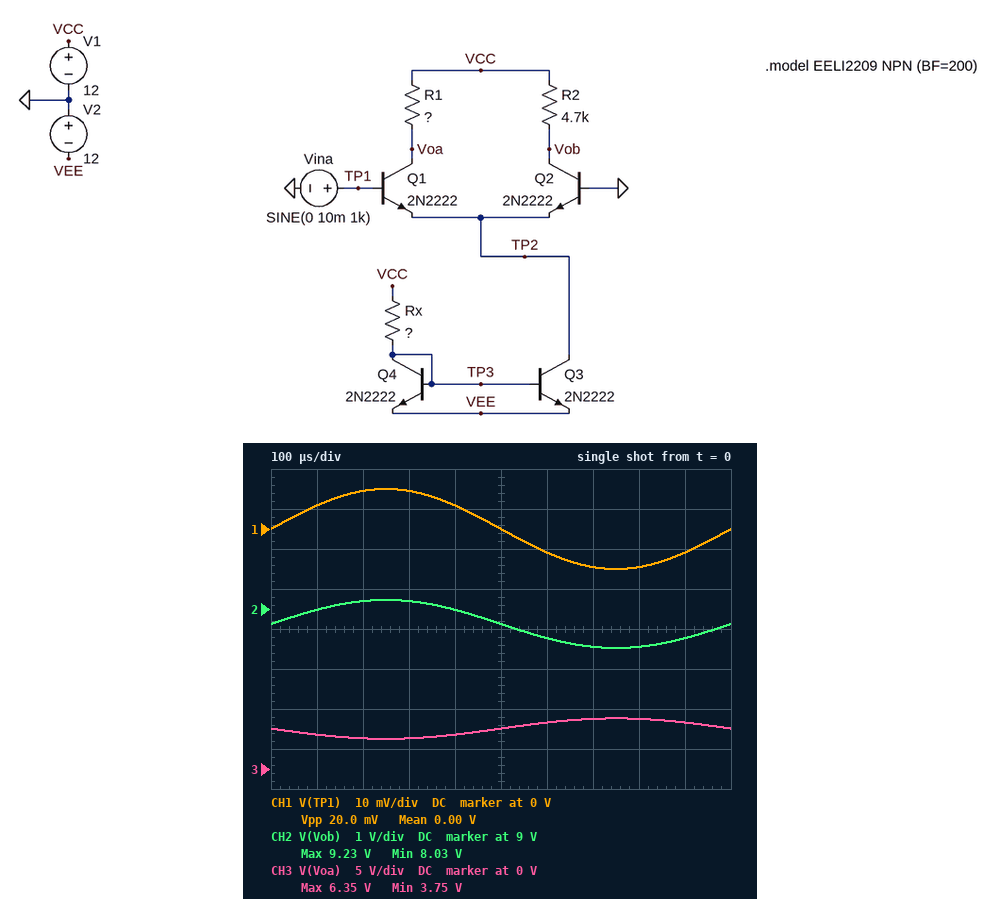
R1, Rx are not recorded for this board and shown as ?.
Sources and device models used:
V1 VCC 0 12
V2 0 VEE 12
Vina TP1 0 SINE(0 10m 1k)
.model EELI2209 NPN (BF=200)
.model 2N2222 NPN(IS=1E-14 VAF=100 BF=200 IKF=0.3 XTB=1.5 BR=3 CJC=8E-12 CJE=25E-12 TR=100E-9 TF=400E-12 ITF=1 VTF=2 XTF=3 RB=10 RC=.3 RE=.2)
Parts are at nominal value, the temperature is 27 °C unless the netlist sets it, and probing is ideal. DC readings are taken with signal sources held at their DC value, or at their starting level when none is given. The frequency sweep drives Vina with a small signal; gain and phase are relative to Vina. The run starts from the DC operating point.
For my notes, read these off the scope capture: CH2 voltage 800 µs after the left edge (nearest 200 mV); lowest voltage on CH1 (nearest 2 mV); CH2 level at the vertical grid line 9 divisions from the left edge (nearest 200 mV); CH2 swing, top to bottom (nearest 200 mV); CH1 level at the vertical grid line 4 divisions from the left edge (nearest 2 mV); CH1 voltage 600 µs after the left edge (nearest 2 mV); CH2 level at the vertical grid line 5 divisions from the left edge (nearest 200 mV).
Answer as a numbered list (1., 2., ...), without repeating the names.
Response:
1. 8.0 V
2. -10 mV
3. 8.2 V
4. 1.2 V
5. 6 mV
6. -6 mV
7. 8.6 V
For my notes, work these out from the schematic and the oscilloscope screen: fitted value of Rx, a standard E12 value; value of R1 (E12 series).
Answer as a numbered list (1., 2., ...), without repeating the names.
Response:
1. 18 kΩ
2. 10 kΩ
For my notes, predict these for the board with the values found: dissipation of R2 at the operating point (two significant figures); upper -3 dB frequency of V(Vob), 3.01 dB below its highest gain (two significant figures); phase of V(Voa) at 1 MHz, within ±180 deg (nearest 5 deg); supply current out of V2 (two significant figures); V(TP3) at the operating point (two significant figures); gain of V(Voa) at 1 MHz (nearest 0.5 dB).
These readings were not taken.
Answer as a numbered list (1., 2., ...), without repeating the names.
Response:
1. 2.4 mW
2. 7.4 MHz
3. 165 deg
4. 2.7 mA
5. -11 V
6. 42.0 dB
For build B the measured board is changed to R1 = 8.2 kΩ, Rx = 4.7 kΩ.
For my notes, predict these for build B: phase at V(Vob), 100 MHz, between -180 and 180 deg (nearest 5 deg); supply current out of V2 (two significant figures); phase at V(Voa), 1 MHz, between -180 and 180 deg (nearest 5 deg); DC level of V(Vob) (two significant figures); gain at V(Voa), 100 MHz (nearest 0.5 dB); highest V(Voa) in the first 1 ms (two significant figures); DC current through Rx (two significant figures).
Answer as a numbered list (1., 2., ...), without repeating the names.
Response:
1. 5 deg
2. 10 mA
3. 25 deg
4. -670 mV
5. -3.5 dB
6. -680 mV
7. 5.0 mA
